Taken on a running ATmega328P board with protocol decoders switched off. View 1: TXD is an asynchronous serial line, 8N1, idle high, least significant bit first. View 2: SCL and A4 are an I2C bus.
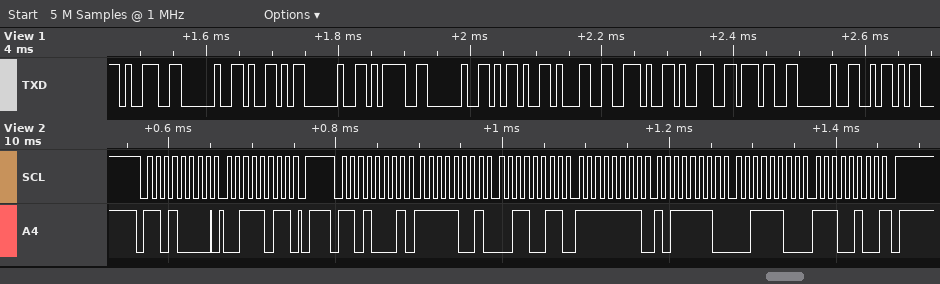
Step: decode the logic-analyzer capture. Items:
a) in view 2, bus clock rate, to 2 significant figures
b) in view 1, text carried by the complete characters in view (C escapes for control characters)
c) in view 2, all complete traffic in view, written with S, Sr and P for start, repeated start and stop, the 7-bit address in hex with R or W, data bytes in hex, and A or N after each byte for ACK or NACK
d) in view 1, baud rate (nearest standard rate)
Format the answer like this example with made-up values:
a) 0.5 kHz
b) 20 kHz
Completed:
a) 100 kHz
b) "9 Y = -1.97 Z"
c) S 68W A 3B A P S 68R A F9 A 33 A FF A BE A 3C A E4 N P
d) 115200 baud
